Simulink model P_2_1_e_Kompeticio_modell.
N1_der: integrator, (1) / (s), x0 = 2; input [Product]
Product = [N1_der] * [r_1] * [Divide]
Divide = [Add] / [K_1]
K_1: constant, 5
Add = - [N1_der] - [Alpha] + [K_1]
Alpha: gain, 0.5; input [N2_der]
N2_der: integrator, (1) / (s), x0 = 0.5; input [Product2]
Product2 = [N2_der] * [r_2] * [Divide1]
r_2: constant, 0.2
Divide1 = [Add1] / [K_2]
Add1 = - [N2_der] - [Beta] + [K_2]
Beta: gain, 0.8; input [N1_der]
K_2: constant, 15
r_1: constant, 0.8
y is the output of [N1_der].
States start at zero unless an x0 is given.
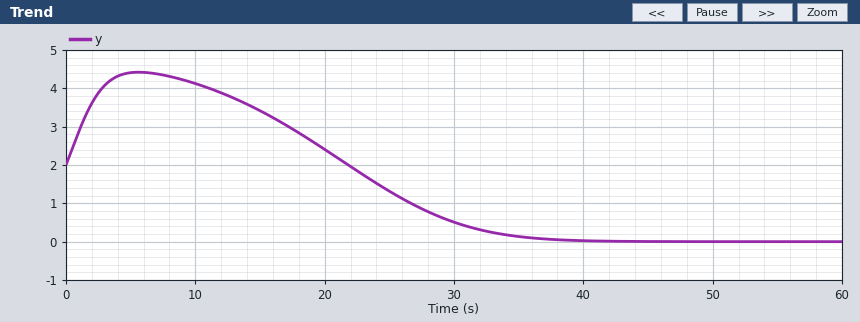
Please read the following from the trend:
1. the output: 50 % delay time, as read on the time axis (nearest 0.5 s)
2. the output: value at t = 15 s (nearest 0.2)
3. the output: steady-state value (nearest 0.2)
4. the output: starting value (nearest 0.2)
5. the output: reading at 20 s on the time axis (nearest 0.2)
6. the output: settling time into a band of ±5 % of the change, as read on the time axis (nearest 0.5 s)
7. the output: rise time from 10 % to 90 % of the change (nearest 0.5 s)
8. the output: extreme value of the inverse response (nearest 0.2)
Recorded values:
26.5 s
3.4
0.0
2.0
2.4
36.0 s
11.0 s
4.4
